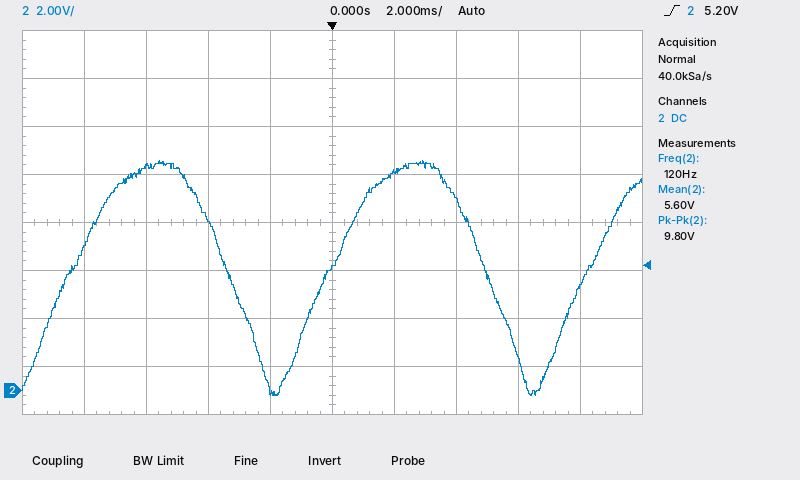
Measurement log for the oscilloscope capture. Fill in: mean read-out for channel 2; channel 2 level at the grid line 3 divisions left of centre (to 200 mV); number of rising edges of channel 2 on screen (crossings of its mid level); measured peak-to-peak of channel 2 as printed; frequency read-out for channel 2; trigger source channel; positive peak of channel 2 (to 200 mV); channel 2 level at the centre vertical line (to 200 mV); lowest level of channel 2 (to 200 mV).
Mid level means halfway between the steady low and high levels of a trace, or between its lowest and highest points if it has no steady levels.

5.60 V
9.4 V
3
9.80 V
120 Hz
channel 2
9.6 V
5.2 V
-200 mV
